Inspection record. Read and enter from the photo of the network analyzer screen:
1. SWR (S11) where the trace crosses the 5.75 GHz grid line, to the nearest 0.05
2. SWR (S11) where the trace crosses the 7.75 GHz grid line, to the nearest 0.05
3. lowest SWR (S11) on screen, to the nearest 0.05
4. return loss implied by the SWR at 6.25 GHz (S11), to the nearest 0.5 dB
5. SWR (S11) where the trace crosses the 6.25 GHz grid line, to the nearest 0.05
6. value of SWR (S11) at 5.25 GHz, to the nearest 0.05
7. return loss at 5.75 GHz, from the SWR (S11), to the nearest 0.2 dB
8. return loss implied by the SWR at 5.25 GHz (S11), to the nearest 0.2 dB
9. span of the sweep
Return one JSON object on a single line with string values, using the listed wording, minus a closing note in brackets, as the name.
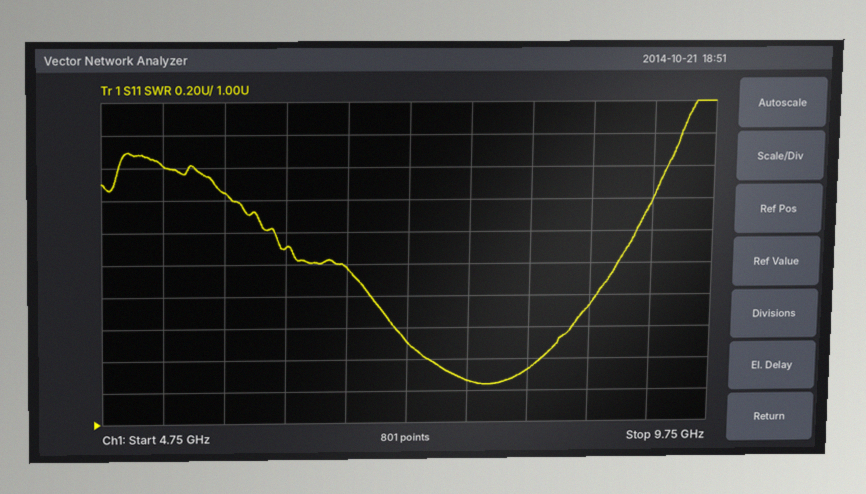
{"SWR (S11) where the trace crosses the 5.75 GHz grid line, to the nearest 0.05": "2.45", "SWR (S11) where the trace crosses the 7.75 GHz grid line, to the nearest 0.05": "1.25", "lowest SWR (S11) on screen, to the nearest 0.05": "1.25", "return loss implied by the SWR at 6.25 GHz (S11), to the nearest 0.5 dB": "9.0 dB", "SWR (S11) where the trace crosses the 6.25 GHz grid line, to the nearest 0.05": "2.10", "value of SWR (S11) at 5.25 GHz, to the nearest 0.05": "2.60", "return loss at 5.75 GHz, from the SWR (S11), to the nearest 0.2 dB": "7.6 dB", "return loss implied by the SWR at 5.25 GHz (S11), to the nearest 0.2 dB": "7.0 dB", "span of the sweep": "5 GHz"}
